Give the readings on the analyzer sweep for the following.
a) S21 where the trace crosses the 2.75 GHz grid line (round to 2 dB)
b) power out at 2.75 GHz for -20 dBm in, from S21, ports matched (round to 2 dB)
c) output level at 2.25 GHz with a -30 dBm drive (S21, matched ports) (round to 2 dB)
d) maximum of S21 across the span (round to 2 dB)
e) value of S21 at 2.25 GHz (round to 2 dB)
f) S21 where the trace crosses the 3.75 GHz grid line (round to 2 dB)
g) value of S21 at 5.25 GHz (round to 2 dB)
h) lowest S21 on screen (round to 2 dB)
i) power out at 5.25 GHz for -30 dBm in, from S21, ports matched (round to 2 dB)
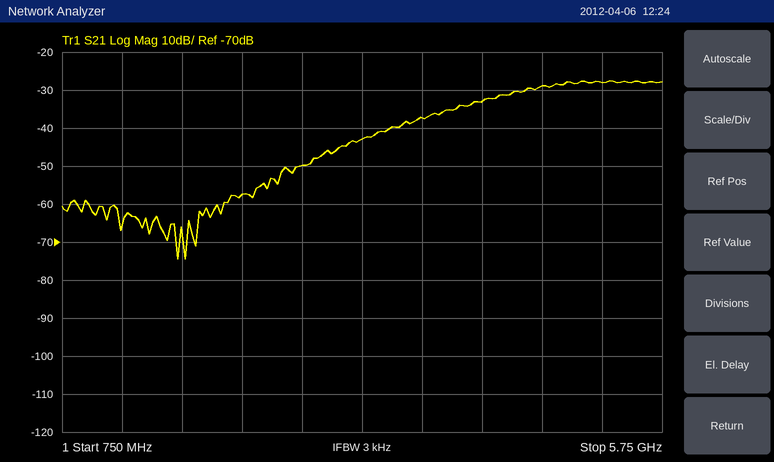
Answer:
-50 dB
-70 dBm
-88 dBm
-28 dB
-58 dB
-38 dB
-28 dB
-74 dB
-58 dBm
